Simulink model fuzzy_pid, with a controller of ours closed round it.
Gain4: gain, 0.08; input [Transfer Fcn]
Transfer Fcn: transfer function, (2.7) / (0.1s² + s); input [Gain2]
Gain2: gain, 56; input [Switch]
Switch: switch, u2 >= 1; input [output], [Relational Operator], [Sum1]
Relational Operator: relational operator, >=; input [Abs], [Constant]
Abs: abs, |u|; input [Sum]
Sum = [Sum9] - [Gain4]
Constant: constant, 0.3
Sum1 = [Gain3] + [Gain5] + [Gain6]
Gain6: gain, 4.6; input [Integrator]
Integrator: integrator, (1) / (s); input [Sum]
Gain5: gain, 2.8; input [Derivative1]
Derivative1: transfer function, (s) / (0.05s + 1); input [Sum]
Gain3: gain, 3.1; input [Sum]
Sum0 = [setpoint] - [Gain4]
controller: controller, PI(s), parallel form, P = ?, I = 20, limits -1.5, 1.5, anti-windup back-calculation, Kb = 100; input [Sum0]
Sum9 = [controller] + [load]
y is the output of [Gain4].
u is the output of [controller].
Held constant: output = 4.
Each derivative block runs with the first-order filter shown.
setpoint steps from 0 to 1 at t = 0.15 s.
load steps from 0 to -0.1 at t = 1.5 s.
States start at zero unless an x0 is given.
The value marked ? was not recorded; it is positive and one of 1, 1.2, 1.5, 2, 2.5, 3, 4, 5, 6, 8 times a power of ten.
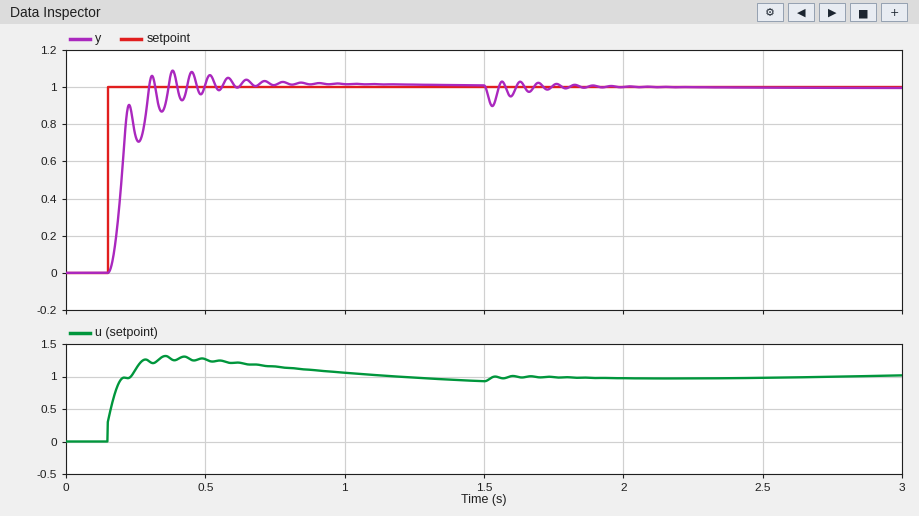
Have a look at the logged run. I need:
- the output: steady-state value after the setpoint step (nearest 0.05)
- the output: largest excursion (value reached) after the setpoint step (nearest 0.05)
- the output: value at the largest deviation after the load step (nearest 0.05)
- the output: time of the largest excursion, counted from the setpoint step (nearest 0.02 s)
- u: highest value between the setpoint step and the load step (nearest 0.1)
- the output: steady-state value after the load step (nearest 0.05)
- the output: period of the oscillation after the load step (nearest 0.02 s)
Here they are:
1.00
1.10
0.90
0.24 s
1.3
1.00
0.06 s
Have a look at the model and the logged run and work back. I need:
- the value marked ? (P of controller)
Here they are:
0.3
